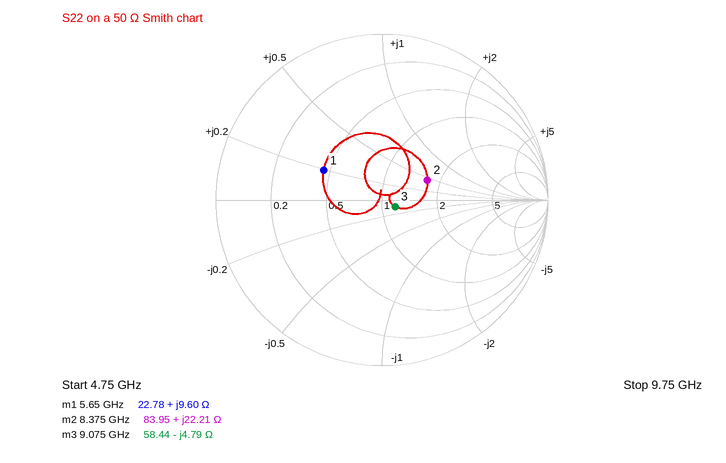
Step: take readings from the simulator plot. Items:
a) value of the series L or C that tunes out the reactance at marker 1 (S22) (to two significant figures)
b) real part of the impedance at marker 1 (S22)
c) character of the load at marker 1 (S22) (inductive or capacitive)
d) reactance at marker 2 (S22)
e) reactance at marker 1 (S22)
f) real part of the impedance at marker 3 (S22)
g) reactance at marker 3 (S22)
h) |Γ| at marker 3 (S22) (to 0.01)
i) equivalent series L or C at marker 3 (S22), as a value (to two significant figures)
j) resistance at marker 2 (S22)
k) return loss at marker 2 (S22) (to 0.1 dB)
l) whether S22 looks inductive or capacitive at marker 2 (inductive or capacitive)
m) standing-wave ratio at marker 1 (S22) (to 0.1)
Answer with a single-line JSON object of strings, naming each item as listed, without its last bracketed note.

{"value of the series L or C that tunes out the reactance at marker 1 (S22)": "2.9 pF", "real part of the impedance at marker 1": "22.78 Ω", "character of the load at marker 1 (S22)": "inductive", "reactance at marker 2": "+22.21 Ω", "reactance at marker 1": "+9.60 Ω", "real part of the impedance at marker 3": "58.44 Ω", "reactance at marker 3": "-4.79 Ω", "|Γ| at marker 3 (S22)": "0.09", "equivalent series L or C at marker 3 (S22), as a value": "3.7 pF", "resistance at marker 2": "83.95 Ω", "return loss at marker 2 (S22)": "10.5 dB", "whether S22 looks inductive or capacitive at marker 2": "inductive", "standing-wave ratio at marker 1 (S22)": "2.3"}
